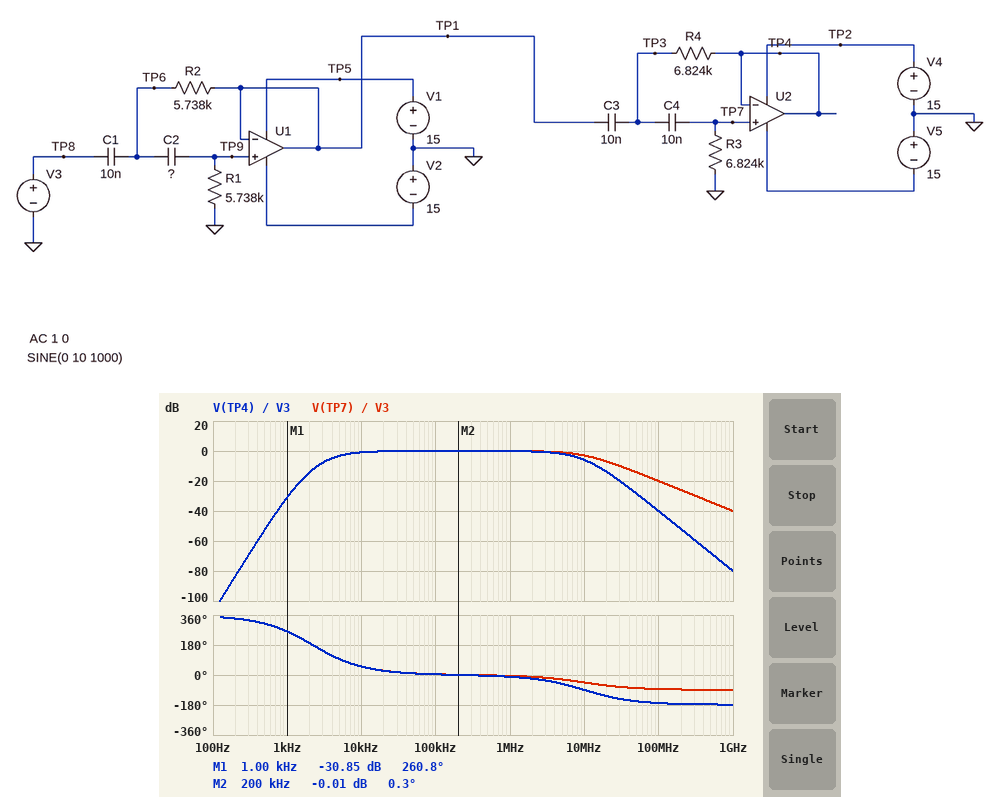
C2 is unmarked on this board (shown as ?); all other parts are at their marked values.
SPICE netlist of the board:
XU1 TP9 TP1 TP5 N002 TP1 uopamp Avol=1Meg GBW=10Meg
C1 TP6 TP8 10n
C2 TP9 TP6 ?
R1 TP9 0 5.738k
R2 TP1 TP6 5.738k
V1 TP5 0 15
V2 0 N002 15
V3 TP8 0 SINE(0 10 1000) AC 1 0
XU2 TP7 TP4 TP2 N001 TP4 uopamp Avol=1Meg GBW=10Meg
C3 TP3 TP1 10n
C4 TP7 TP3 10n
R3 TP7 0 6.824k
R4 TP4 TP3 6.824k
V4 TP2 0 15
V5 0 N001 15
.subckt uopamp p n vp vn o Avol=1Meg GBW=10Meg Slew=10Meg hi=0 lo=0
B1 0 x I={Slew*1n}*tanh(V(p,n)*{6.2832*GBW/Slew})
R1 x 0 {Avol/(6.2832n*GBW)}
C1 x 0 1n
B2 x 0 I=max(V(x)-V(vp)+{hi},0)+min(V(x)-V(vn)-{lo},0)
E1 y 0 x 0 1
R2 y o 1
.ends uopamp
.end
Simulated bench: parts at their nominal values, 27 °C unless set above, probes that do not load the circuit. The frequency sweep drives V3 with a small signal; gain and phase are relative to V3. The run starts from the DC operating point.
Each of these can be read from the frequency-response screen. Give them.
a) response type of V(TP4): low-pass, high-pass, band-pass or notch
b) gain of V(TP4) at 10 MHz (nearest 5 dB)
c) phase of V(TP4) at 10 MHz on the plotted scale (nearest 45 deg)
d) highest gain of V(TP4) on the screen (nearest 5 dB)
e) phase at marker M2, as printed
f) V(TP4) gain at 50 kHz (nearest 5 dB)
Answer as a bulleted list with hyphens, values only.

- band-pass
- -5 dB
- -90 deg
- 0 dB
- 0.3 deg
- 0 dB
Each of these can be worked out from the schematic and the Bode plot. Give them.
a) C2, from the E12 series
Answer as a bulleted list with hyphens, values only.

- 18 nF
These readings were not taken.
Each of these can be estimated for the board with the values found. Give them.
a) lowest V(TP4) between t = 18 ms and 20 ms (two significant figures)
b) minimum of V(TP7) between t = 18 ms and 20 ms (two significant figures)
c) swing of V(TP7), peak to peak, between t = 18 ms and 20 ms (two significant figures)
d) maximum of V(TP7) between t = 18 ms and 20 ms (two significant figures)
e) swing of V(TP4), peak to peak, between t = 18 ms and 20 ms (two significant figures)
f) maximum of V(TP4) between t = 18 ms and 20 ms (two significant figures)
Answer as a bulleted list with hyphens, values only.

- -290 mV
- -290 mV
- 570 mV
- 290 mV
- 570 mV
- 290 mV
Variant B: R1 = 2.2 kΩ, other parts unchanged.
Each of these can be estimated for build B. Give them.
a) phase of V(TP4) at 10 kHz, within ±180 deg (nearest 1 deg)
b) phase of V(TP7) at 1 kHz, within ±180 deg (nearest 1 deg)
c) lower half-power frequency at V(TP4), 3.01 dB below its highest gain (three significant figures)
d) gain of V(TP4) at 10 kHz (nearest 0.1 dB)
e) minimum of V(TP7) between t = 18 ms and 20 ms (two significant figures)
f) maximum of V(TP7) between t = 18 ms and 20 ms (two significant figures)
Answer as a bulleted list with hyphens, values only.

- 78 deg
- -94 deg
- 11.2 kHz
- -3.6 dB
- -100 mV
- 100 mV
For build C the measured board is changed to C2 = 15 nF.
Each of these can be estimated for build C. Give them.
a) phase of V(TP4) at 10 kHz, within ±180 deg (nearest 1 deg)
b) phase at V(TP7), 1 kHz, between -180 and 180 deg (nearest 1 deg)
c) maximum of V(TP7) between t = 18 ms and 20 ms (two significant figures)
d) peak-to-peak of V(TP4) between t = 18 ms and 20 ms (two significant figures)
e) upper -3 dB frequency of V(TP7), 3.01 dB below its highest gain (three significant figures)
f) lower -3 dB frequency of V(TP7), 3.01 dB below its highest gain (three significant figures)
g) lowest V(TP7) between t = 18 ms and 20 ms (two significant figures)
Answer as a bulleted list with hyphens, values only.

- 52 deg
- -95 deg
- 250 mV
- 500 mV
- 10.0 MHz
- 5.37 kHz
- -250 mV
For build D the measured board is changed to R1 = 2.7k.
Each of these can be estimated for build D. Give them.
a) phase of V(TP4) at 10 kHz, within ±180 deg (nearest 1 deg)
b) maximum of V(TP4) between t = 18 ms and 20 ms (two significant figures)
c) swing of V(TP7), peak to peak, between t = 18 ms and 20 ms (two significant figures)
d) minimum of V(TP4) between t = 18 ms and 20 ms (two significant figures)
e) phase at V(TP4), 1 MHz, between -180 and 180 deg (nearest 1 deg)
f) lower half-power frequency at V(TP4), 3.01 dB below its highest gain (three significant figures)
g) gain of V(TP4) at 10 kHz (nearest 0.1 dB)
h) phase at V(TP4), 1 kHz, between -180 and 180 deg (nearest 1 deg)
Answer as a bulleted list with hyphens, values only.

- 71 deg
- 130 mV
- 250 mV
- -130 mV
- -11 deg
- 9.29 kHz
- -2.7 dB
- -95 deg
